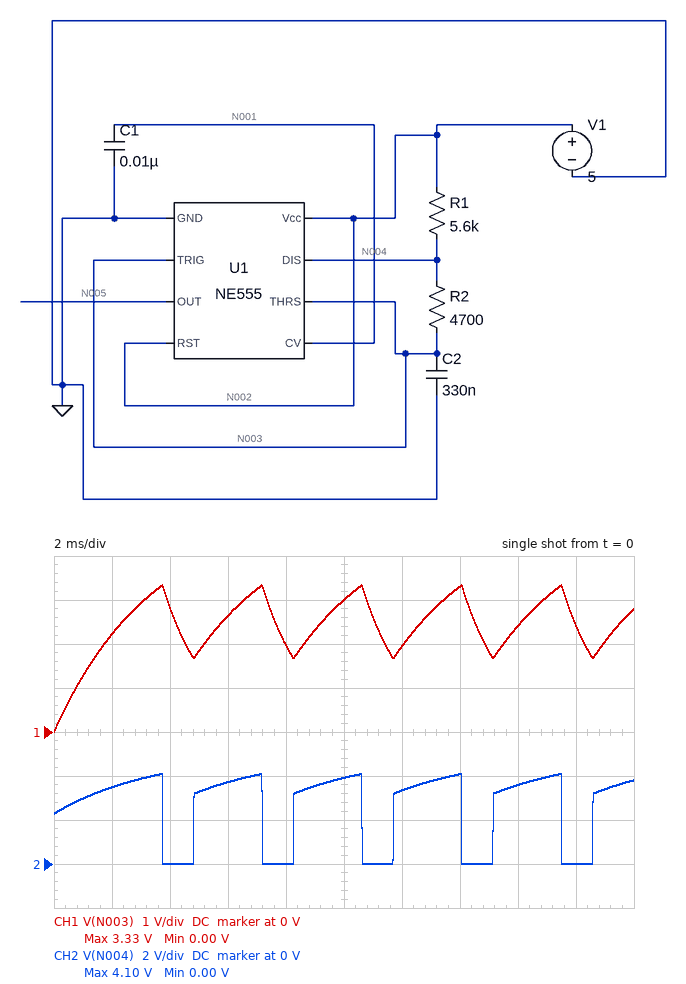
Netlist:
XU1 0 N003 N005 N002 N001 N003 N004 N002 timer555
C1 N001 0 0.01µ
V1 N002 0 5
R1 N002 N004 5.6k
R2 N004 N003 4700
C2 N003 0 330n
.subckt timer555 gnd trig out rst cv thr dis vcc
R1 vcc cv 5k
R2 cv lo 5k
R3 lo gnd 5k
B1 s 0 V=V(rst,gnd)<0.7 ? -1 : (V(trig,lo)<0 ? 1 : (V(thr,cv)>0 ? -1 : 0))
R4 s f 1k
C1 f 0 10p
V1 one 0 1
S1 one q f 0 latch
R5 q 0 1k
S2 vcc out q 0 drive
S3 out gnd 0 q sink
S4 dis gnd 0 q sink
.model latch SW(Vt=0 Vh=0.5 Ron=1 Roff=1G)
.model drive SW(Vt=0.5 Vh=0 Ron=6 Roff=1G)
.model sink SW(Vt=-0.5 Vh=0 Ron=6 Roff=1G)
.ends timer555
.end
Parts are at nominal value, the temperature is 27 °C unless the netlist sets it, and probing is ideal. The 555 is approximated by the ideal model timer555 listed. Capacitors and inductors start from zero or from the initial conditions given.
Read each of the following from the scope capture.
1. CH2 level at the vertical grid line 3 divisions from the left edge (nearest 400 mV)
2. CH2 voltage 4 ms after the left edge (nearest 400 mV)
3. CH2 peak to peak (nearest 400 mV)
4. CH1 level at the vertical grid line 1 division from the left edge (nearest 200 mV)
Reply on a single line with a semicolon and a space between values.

3.6 V; 0 V; 4.0 V; 2.2 V
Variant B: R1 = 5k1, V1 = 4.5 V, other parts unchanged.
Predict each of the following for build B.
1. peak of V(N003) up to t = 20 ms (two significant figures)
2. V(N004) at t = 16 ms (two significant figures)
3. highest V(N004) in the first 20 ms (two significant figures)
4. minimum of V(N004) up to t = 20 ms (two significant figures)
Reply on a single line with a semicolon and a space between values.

3.0 V; 3.5 V; 3.7 V; 7.2 mV
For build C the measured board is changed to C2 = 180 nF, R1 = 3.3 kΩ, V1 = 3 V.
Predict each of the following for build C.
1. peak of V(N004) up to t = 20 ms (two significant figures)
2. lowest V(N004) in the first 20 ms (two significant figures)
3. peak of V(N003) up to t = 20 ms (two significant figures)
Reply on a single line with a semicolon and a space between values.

2.6 V; 6.7 mV; 2.0 V
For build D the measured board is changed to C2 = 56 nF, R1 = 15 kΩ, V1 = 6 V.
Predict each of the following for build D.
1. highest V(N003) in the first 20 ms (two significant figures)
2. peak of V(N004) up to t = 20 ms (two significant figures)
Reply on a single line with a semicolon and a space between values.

4.0 V; 4.5 V
